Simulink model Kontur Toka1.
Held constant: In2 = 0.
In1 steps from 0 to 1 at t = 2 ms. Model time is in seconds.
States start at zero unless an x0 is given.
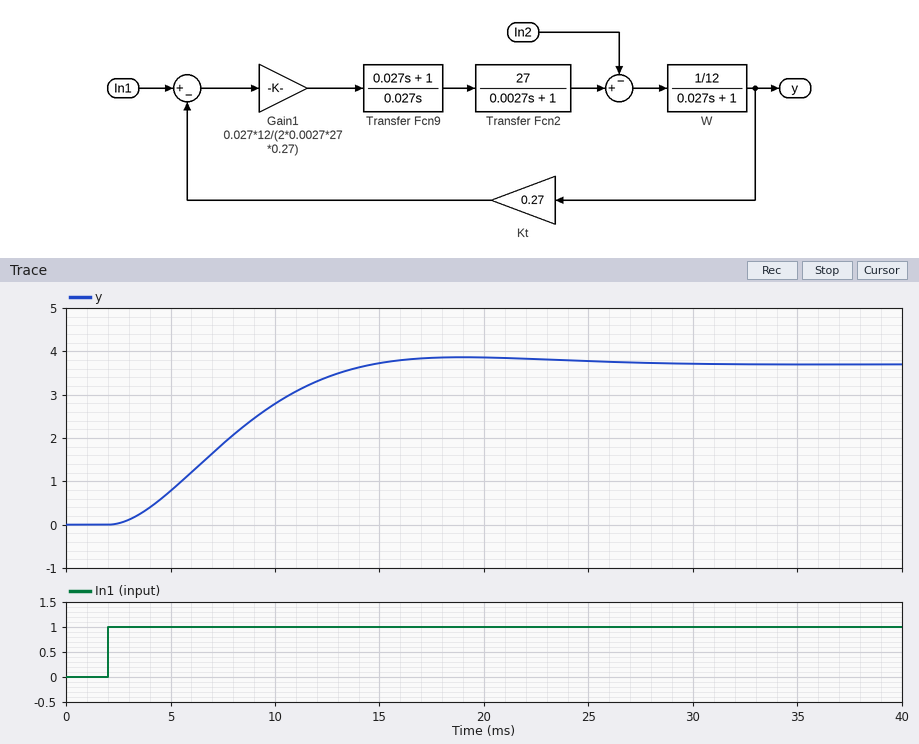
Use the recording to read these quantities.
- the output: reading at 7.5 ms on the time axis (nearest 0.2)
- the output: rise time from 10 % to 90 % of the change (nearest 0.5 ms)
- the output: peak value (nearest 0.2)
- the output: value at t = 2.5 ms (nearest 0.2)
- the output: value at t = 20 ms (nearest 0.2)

1.8
8.0 ms
3.8
0.0
3.8
